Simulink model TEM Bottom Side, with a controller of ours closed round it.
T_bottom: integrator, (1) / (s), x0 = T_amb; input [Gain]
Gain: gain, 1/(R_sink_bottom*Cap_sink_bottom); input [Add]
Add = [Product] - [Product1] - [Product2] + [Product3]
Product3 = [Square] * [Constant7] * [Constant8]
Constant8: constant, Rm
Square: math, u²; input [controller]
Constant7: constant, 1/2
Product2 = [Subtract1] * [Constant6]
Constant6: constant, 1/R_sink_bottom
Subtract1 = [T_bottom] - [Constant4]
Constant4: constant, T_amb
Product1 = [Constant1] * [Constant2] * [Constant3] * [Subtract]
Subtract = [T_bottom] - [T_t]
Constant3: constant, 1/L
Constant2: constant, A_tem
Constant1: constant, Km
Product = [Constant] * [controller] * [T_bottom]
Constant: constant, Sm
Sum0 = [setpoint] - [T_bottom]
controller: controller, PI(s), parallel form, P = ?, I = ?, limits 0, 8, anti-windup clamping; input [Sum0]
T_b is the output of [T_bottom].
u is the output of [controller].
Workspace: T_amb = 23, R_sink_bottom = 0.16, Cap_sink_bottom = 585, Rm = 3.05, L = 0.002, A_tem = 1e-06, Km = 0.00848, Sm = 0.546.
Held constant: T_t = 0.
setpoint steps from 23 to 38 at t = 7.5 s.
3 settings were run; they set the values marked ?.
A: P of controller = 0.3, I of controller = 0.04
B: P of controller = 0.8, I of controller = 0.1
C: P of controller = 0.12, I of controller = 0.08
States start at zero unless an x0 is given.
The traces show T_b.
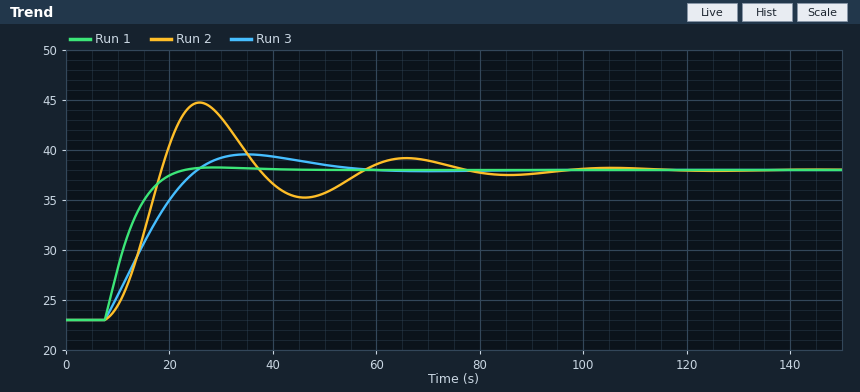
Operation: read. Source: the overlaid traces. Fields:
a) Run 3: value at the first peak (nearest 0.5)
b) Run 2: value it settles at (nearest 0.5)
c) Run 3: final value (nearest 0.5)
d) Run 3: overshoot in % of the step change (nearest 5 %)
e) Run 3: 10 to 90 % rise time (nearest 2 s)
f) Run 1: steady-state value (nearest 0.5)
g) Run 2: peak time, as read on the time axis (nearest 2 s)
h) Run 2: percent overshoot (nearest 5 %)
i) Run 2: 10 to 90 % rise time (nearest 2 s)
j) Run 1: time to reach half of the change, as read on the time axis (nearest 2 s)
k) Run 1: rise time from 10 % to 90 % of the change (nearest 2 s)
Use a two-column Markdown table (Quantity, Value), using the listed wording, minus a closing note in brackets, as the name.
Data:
| Quantity | Value |
|---|---|
| Run 3: value at the first peak | 39.5 |
| Run 2: value it settles at | 38.0 |
| Run 3: final value | 38.0 |
| Run 3: overshoot in % of the step change | 10 % |
| Run 3: 10 to 90 % rise time | 14 s |
| Run 1: steady-state value | 38.0 |
| Run 2: peak time, as read on the time axis | 26 s |
| Run 2: percent overshoot | 45 % |
| Run 2: 10 to 90 % rise time | 8 s |
| Run 1: time to reach half of the change, as read on the time axis | 12 s |
| Run 1: rise time from 10 % to 90 % of the change | 10 s |
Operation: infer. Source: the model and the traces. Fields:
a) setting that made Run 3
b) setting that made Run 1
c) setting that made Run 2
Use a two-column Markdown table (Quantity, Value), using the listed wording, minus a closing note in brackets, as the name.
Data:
| Quantity | Value |
|---|---|
| setting that made Run 3 | A |
| setting that made Run 1 | B |
| setting that made Run 2 | C |
